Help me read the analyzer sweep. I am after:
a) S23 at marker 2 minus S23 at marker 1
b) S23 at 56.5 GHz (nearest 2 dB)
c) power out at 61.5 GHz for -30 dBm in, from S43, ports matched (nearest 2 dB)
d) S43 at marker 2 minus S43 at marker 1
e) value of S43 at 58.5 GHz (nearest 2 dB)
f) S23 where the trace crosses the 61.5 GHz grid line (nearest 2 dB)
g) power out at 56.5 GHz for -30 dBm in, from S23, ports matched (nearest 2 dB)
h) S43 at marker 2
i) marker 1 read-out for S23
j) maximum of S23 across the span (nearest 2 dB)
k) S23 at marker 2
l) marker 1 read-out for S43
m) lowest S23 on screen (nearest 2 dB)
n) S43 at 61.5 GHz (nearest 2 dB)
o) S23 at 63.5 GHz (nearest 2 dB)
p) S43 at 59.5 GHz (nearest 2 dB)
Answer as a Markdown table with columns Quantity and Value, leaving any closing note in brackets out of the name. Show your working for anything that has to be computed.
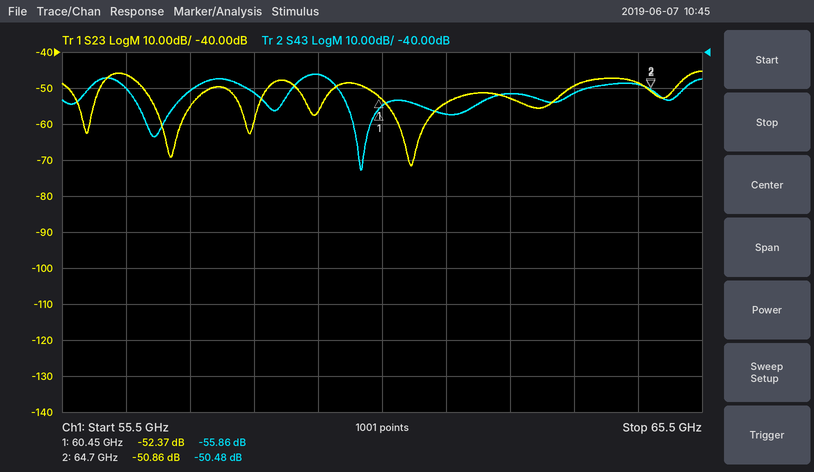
| Quantity | Value |
|---|---|
| S23 at marker 2 minus S23 at marker 1 | -50.86 − (-52.37) = 1.51 dB |
| S23 at 56.5 GHz | -46 dB |
| power out at 61.5 GHz for -30 dBm in, from S43, ports matched | -30 dBm + (-58 dB) = -88 dBm |
| S43 at marker 2 minus S43 at marker 1 | -50.48 − (-55.86) = 5.38 dB |
| value of S43 at 58.5 GHz | -52 dB |
| S23 where the trace crosses the 61.5 GHz grid line | -54 dB |
| power out at 56.5 GHz for -30 dBm in, from S23, ports matched | -30 dBm + (-46 dB) = -76 dBm |
| S43 at marker 2 | -50.48 dB |
| marker 1 read-out for S23 | -52.37 dB |
| maximum of S23 across the span | -46 dB |
| S23 at marker 2 | -50.86 dB |
| marker 1 read-out for S43 | -55.86 dB |
| lowest S23 on screen | -72 dB |
| S43 at 61.5 GHz | -58 dB |
| S23 at 63.5 GHz | -50 dB |
| S43 at 59.5 GHz | -46 dB |
